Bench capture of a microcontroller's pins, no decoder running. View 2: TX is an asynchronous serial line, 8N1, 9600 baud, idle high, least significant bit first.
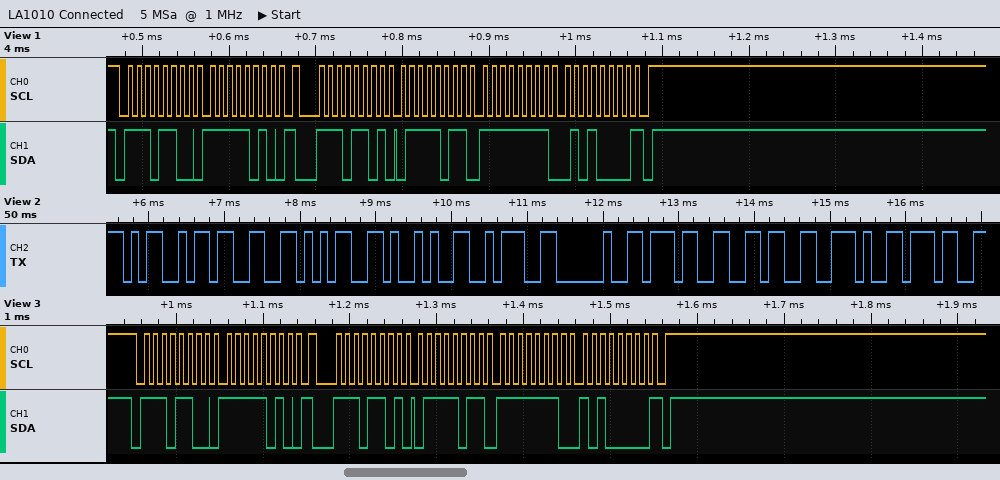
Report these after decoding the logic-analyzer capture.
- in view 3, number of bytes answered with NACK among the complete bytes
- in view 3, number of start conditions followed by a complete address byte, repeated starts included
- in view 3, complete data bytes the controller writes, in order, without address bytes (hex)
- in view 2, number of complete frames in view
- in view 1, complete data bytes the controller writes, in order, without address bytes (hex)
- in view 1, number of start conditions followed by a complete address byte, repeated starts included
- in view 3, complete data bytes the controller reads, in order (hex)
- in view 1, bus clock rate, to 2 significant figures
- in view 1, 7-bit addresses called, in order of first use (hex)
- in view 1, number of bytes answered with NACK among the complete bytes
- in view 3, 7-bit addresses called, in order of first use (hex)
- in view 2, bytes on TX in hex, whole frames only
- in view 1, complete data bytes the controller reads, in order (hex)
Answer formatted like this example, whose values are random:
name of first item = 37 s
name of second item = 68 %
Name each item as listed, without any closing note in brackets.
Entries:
in view 3, number of bytes answered with NACK among the complete bytes = 1
in view 3, number of start conditions followed by a complete address byte, repeated starts included = 2
in view 3, complete data bytes the controller writes, in order, without address bytes = FA
in view 2, number of complete frames in view = 10
in view 1, complete data bytes the controller writes, in order, without address bytes = FA
in view 1, number of start conditions followed by a complete address byte, repeated starts included = 2
in view 3, complete data bytes the controller reads, in order = 7B FE A0
in view 1, bus clock rate, to 2 significant figures = 100 kHz
in view 1, 7-bit addresses called, in order of first use = 0x76
in view 1, number of bytes answered with NACK among the complete bytes = 1
in view 3, 7-bit addresses called, in order of first use = 0x76
in view 2, bytes on TX in hex, whole frames only = 4D 33 35 29 3A 20 37 36 2E 37
in view 1, complete data bytes the controller reads, in order = 7B FF 50
